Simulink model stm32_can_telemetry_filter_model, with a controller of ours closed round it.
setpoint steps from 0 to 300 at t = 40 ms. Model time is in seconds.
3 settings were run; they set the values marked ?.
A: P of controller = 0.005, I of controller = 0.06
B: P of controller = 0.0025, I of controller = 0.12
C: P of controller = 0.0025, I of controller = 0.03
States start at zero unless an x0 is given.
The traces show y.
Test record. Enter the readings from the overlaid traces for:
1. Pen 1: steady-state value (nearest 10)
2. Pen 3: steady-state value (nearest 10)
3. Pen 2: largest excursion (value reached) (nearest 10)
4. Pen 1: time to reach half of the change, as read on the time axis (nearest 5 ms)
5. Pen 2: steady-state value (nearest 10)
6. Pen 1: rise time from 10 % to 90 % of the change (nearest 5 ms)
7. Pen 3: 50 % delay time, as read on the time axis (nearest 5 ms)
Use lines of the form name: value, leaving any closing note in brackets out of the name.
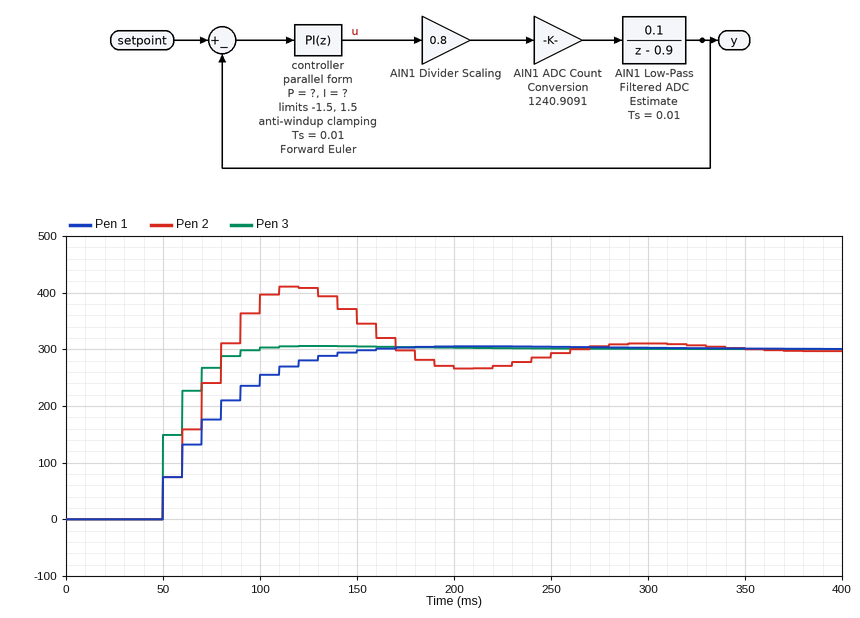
Pen 1: steady-state value: 300
Pen 3: steady-state value: 300
Pen 2: largest excursion (value reached): 410
Pen 1: time to reach half of the change, as read on the time axis: 70 ms
Pen 2: steady-state value: 300
Pen 1: rise time from 10 % to 90 % of the change: 70 ms
Pen 3: 50 % delay time, as read on the time axis: 60 ms
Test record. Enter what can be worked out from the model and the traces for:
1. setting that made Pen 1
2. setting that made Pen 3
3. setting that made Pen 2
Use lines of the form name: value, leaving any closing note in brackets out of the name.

setting that made Pen 1: C
setting that made Pen 3: A
setting that made Pen 2: B
